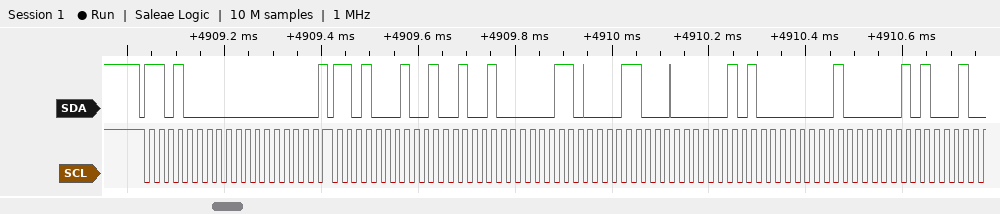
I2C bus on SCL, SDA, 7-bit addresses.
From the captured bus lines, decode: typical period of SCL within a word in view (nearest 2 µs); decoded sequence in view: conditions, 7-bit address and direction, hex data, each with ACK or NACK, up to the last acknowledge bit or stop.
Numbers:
20 µs
start, address 68 write ACK, 00 ACK, repeated start, address 68 read ACK, 49 ACK, 06 ACK, 18 ACK, 05 ACK, 01 ACK, 05 ACK
